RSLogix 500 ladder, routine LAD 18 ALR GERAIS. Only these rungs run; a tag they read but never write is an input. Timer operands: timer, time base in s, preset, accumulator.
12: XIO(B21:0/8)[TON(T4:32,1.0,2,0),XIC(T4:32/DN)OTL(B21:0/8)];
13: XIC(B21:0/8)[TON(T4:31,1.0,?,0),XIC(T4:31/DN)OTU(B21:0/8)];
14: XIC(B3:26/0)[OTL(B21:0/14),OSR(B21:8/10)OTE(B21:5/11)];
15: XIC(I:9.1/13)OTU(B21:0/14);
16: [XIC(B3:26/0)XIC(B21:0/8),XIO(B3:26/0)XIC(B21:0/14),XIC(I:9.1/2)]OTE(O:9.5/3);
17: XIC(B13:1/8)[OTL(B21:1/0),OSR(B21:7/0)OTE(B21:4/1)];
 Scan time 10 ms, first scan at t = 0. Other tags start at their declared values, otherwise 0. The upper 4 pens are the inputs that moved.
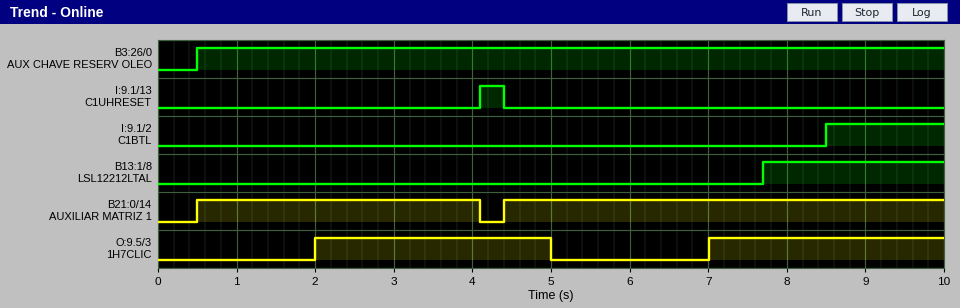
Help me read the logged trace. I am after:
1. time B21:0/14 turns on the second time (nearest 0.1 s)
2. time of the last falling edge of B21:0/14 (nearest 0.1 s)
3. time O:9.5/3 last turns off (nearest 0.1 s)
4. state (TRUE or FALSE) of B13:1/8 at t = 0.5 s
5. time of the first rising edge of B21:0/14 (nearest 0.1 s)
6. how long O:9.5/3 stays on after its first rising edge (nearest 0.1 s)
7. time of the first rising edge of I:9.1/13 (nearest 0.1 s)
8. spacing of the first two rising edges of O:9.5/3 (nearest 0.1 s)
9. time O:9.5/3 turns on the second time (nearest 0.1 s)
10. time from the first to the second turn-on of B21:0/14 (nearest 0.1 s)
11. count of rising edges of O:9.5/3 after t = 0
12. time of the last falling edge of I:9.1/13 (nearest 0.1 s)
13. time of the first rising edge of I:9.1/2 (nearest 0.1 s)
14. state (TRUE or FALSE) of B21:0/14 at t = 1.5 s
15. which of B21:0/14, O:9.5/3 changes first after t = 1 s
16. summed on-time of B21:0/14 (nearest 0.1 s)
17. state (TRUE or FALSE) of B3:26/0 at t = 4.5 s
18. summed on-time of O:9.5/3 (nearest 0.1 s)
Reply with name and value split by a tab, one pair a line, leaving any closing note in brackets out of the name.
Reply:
time B21:0/14 turns on the second time	4.4 s
time of the last falling edge of B21:0/14	4.1 s
time O:9.5/3 last turns off	5.0 s
state (TRUE or FALSE) of B13:1/8 at t = 0.5 s	FALSE
time of the first rising edge of B21:0/14	0.5 s
how long O:9.5/3 stays on after its first rising edge	3.0 s
time of the first rising edge of I:9.1/13	4.1 s
spacing of the first two rising edges of O:9.5/3	5.0 s
time O:9.5/3 turns on the second time	7.0 s
time from the first to the second turn-on of B21:0/14	3.9 s
count of rising edges of O:9.5/3 after t = 0	2
time of the last falling edge of I:9.1/13	4.4 s
time of the first rising edge of I:9.1/2	8.5 s
state (TRUE or FALSE) of B21:0/14 at t = 1.5 s	TRUE
which of B21:0/14, O:9.5/3 changes first after t = 1 s	O:9.5/3
summed on-time of B21:0/14	9.2 s
state (TRUE or FALSE) of B3:26/0 at t = 4.5 s	TRUE
summed on-time of O:9.5/3	6.0 s
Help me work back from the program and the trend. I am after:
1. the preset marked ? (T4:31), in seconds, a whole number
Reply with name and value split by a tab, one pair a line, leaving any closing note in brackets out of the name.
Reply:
the preset marked ? (T4:31), in seconds, a whole number	3 s
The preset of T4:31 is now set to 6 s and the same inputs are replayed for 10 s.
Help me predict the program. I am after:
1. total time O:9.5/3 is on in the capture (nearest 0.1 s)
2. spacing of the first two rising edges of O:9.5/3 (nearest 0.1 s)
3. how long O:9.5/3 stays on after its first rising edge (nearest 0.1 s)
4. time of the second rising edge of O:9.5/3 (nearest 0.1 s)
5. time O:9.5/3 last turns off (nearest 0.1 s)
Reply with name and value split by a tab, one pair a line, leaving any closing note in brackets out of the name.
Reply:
total time O:9.5/3 is on in the capture	7.5 s
spacing of the first two rising edges of O:9.5/3	6.5 s
how long O:9.5/3 stays on after its first rising edge	6.0 s
time of the second rising edge of O:9.5/3	8.5 s
time O:9.5/3 last turns off	8.0 s
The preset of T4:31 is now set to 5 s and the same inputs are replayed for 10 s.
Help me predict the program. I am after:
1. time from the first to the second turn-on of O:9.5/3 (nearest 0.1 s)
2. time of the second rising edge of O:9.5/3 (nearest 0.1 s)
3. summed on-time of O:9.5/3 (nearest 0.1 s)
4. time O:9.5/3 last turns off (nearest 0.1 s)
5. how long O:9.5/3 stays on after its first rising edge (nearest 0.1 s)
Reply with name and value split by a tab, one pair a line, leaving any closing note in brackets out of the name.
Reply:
time from the first to the second turn-on of O:9.5/3	6.5 s
time of the second rising edge of O:9.5/3	8.5 s
summed on-time of O:9.5/3	6.5 s
time O:9.5/3 last turns off	7.0 s
how long O:9.5/3 stays on after its first rising edge	5.0 s
